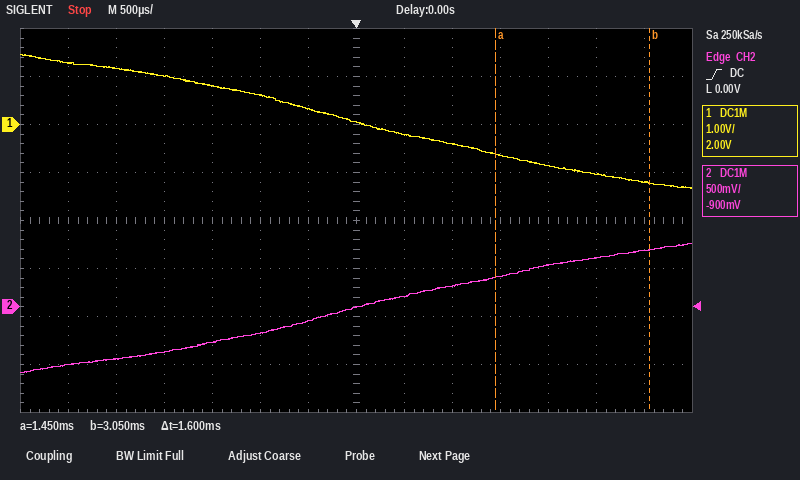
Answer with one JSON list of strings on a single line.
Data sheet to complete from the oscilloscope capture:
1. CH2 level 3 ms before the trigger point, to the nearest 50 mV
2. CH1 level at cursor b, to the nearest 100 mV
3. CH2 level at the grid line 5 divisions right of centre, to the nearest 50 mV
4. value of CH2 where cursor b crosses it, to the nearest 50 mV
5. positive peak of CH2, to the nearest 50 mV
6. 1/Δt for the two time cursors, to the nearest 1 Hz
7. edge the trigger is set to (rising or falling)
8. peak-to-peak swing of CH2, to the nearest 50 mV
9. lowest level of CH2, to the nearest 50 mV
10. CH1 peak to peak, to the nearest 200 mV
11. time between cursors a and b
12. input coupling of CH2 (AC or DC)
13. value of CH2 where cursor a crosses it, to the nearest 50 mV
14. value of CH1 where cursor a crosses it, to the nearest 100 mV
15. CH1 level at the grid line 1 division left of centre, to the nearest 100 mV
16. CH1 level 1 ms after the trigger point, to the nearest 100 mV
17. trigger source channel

["-600 mV", "-1.2 V", "500 mV", "600 mV", "650 mV", "625 Hz", "rising", "1.35 V", "-700 mV", "2.8 V", "1.6 ms", "DC", "300 mV", "-600 mV", "300 mV", "-400 mV", "CH2"]
